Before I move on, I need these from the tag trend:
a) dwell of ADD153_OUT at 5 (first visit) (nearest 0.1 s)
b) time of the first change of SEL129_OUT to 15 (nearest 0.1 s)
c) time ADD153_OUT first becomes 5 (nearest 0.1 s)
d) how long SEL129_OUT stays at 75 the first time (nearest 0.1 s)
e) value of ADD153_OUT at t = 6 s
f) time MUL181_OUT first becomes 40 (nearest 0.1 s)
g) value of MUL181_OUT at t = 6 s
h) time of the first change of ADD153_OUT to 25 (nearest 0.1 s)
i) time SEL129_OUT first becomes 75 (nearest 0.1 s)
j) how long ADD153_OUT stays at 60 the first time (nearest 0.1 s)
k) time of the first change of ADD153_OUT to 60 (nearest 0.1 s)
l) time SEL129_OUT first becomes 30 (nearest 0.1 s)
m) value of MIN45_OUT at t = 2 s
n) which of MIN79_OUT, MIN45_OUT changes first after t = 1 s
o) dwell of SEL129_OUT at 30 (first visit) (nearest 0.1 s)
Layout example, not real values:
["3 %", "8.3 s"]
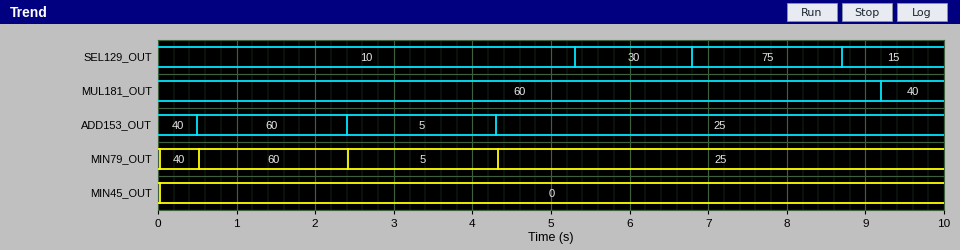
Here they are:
["1.9 s", "8.7 s", "2.4 s", "1.9 s", "25", "9.2 s", "60", "4.3 s", "6.8 s", "1.9 s", "0.5 s", "5.3 s", "0", "MIN79_OUT", "1.5 s"]
